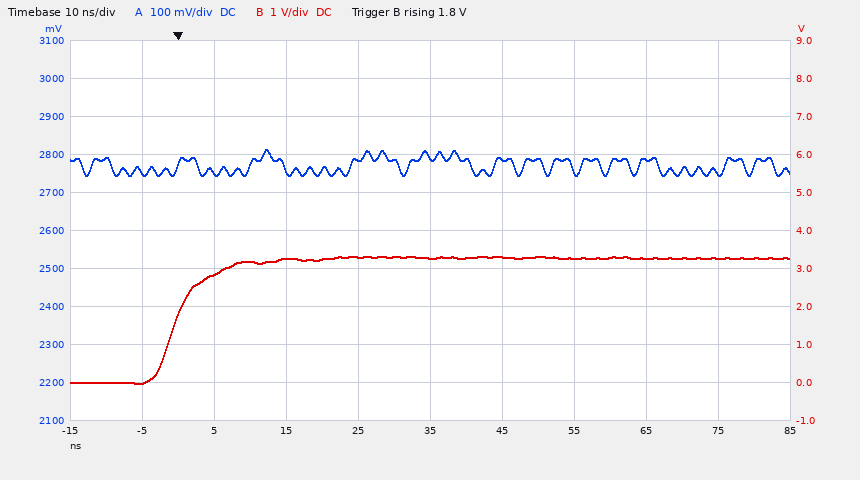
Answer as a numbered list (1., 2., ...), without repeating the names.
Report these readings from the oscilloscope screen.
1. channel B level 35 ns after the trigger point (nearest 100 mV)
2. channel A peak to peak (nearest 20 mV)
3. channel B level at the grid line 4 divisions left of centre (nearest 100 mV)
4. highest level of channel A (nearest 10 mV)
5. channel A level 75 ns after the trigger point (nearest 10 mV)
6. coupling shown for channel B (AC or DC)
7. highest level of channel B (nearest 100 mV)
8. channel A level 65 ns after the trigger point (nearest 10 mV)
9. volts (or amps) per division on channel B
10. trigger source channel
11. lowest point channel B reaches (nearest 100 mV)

1. 3.3 V
2. 60 mV
3. 0.0 V
4. 2.81 V
5. 2.75 V
6. DC
7. 3.3 V
8. 2.79 V
9. 1 V
10. channel B
11. 0.0 V
